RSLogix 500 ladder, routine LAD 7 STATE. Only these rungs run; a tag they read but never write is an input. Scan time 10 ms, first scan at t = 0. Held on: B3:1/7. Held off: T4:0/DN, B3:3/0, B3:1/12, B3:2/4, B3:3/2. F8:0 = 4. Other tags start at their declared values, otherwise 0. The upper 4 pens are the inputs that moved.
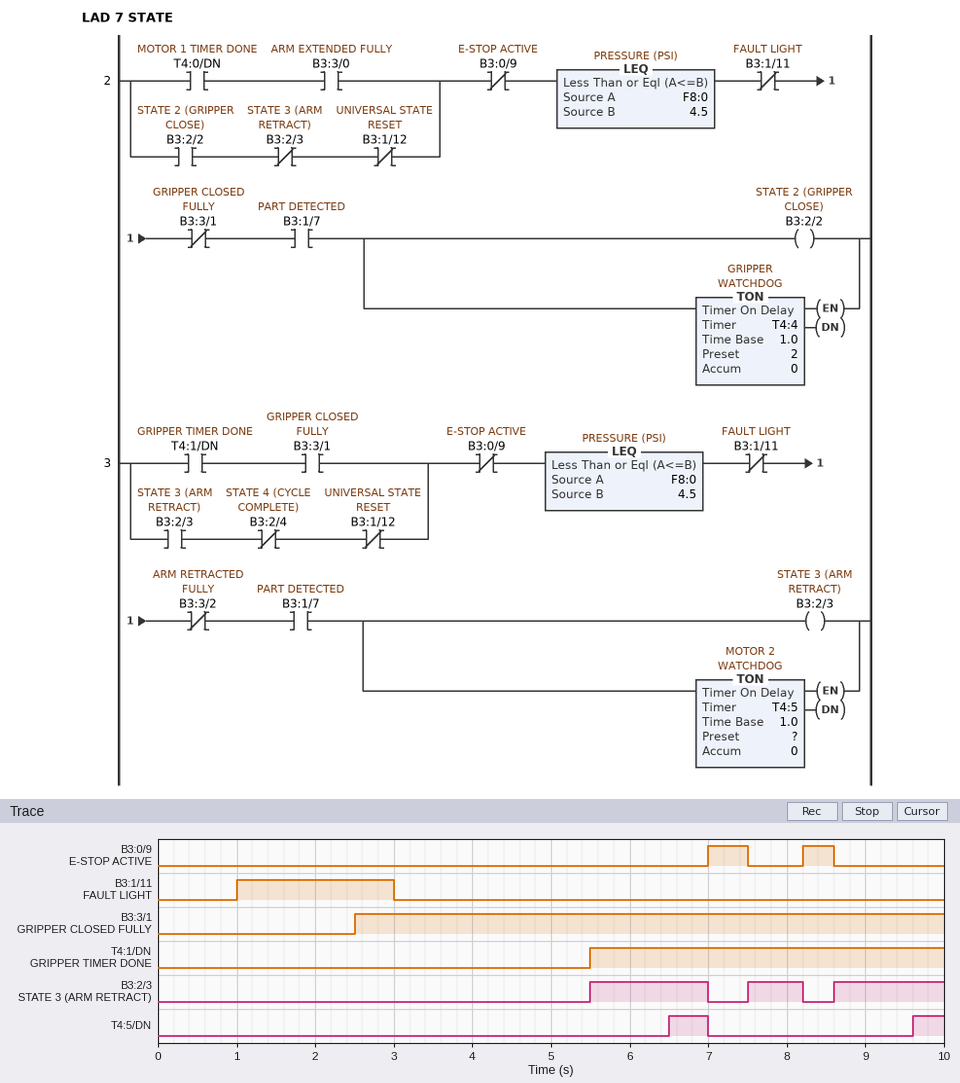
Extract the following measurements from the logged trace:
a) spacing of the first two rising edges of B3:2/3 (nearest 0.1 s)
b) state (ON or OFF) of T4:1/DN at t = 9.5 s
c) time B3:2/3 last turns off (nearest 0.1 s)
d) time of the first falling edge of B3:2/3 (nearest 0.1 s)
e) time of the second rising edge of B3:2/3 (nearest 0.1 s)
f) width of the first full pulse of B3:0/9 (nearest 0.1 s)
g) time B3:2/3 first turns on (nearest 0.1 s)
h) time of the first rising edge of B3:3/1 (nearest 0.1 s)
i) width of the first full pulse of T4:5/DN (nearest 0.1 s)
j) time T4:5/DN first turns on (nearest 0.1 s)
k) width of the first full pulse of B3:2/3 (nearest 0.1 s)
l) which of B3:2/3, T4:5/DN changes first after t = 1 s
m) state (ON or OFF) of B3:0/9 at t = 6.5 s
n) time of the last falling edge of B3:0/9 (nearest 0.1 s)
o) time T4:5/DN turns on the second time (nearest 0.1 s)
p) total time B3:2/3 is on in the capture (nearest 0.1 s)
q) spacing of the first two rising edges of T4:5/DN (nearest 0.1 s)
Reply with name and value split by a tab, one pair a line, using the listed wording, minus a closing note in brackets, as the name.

spacing of the first two rising edges of B3:2/3	2.0 s
state (ON or OFF) of T4:1/DN at t = 9.5 s	ON
time B3:2/3 last turns off	8.2 s
time of the first falling edge of B3:2/3	7.0 s
time of the second rising edge of B3:2/3	7.5 s
width of the first full pulse of B3:0/9	0.5 s
time B3:2/3 first turns on	5.5 s
time of the first rising edge of B3:3/1	2.5 s
width of the first full pulse of T4:5/DN	0.5 s
time T4:5/DN first turns on	6.5 s
width of the first full pulse of B3:2/3	1.5 s
which of B3:2/3, T4:5/DN changes first after t = 1 s	B3:2/3
state (ON or OFF) of B3:0/9 at t = 6.5 s	OFF
time of the last falling edge of B3:0/9	8.6 s
time T4:5/DN turns on the second time	9.6 s
total time B3:2/3 is on in the capture	3.6 s
spacing of the first two rising edges of T4:5/DN	3.1 s
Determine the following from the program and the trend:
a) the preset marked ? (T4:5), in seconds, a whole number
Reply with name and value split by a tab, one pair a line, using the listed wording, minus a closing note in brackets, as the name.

the preset marked ? (T4:5), in seconds, a whole number	1 s
